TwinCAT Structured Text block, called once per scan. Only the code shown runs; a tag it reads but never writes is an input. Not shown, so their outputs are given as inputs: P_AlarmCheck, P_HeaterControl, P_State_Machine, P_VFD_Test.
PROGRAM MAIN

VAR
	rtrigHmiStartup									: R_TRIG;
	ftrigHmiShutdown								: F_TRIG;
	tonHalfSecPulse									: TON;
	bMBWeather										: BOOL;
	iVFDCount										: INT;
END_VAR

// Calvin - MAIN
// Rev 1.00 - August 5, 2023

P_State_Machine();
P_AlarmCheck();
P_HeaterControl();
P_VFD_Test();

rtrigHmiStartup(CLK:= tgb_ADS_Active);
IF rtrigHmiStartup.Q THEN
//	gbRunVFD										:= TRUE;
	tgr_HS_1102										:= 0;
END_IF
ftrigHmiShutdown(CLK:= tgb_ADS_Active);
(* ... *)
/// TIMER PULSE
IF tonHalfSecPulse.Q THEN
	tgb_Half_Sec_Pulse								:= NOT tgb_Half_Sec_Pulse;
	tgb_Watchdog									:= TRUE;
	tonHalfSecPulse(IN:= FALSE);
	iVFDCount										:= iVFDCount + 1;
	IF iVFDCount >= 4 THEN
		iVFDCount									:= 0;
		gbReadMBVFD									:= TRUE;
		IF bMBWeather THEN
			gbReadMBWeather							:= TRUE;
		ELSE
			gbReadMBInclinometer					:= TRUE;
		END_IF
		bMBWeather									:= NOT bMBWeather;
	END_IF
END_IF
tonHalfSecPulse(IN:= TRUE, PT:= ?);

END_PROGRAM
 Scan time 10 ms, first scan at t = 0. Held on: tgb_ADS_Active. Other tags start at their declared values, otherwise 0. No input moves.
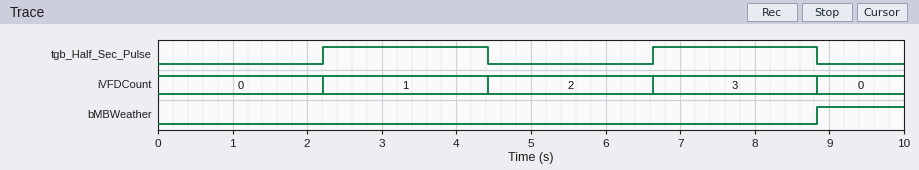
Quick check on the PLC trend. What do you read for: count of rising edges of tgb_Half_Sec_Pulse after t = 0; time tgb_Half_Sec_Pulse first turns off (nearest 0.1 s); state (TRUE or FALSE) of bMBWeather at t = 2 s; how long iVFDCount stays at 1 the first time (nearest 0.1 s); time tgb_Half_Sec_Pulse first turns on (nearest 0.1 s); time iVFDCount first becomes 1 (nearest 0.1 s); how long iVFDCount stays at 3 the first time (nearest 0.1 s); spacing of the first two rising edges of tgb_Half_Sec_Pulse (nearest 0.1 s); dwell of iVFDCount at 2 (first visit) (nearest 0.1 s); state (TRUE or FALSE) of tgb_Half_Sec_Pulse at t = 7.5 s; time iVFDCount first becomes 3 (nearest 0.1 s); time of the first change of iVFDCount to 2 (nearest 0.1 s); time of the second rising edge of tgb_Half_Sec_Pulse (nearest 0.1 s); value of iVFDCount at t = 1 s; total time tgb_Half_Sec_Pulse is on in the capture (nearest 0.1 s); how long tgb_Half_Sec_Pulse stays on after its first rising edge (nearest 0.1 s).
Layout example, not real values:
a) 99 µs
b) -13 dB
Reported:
a) 2
b) 4.4 s
c) FALSE
d) 2.2 s
e) 2.2 s
f) 2.2 s
g) 2.2 s
h) 4.4 s
i) 2.2 s
j) TRUE
k) 6.6 s
l) 4.4 s
m) 6.6 s
n) 0
o) 4.4 s
p) 2.2 s
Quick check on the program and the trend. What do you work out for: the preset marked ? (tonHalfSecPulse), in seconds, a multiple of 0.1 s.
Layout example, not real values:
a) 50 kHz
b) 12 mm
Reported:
a) 2.2 s
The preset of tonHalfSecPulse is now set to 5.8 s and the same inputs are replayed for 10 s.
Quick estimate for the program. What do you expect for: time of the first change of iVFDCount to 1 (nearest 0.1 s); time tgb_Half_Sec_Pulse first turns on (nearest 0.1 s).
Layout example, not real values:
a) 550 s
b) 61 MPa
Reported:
a) 5.8 s
b) 5.8 s
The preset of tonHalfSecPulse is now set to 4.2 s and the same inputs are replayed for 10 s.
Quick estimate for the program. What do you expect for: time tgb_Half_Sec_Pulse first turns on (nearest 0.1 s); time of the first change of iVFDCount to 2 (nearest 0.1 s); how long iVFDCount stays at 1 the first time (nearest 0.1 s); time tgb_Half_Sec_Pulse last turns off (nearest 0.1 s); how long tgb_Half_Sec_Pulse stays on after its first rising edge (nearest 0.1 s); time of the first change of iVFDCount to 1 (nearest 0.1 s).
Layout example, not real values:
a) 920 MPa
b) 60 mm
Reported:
a) 4.2 s
b) 8.4 s
c) 4.2 s
d) 8.4 s
e) 4.2 s
f) 4.2 s
